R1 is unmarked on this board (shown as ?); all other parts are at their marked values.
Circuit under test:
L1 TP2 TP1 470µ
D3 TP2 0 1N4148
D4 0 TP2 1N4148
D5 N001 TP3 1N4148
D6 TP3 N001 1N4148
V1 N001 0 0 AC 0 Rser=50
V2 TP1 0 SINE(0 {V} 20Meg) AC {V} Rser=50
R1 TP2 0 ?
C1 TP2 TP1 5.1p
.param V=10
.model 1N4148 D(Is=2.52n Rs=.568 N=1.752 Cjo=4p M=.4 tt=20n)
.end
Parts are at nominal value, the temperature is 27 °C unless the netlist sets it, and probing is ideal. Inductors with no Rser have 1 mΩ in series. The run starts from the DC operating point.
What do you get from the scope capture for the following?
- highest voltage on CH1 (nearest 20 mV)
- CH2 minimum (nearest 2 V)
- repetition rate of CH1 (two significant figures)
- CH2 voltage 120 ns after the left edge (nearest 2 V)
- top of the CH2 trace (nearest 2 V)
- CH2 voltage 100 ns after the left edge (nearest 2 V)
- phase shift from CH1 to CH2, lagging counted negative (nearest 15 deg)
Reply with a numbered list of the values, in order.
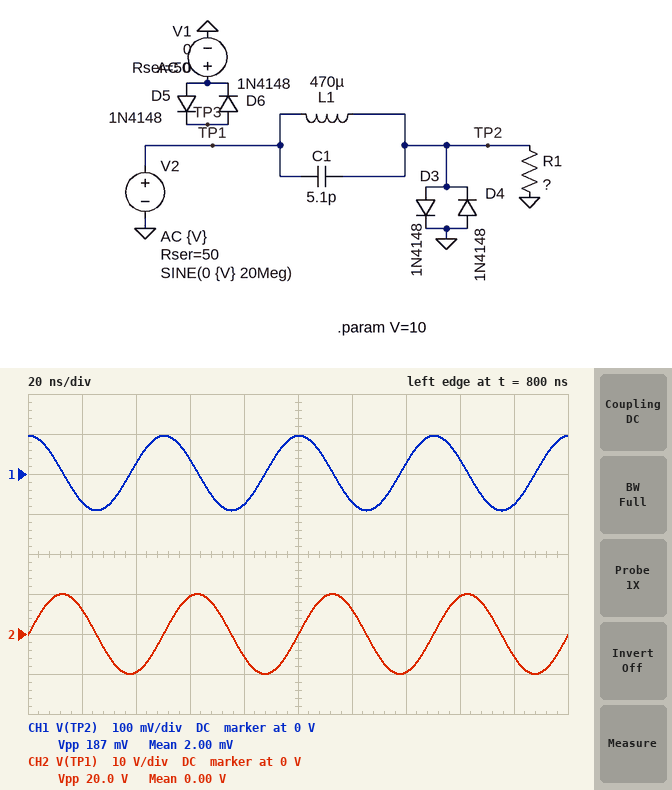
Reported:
1. 100 mV
2. -10 V
3. 20 MHz
4. 6 V
5. 10 V
6. 0 V
7. -90 deg
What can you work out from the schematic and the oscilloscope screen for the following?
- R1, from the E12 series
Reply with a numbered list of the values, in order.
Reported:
1. 15 Ω
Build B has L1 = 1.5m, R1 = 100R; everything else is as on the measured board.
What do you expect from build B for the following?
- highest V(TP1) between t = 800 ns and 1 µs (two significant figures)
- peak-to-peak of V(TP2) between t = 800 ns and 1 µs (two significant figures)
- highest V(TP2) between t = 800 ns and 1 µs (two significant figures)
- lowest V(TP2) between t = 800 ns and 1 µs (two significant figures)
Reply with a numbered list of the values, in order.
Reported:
1. 10 V
2. 1.1 V
3. 530 mV
4. -530 mV
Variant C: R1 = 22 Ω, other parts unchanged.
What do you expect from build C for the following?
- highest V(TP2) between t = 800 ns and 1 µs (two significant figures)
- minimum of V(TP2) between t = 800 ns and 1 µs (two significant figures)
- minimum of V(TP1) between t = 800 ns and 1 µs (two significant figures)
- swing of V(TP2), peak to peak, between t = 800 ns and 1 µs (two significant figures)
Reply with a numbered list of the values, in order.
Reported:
1. 140 mV
2. -130 mV
3. -10 V
4. 270 mV
